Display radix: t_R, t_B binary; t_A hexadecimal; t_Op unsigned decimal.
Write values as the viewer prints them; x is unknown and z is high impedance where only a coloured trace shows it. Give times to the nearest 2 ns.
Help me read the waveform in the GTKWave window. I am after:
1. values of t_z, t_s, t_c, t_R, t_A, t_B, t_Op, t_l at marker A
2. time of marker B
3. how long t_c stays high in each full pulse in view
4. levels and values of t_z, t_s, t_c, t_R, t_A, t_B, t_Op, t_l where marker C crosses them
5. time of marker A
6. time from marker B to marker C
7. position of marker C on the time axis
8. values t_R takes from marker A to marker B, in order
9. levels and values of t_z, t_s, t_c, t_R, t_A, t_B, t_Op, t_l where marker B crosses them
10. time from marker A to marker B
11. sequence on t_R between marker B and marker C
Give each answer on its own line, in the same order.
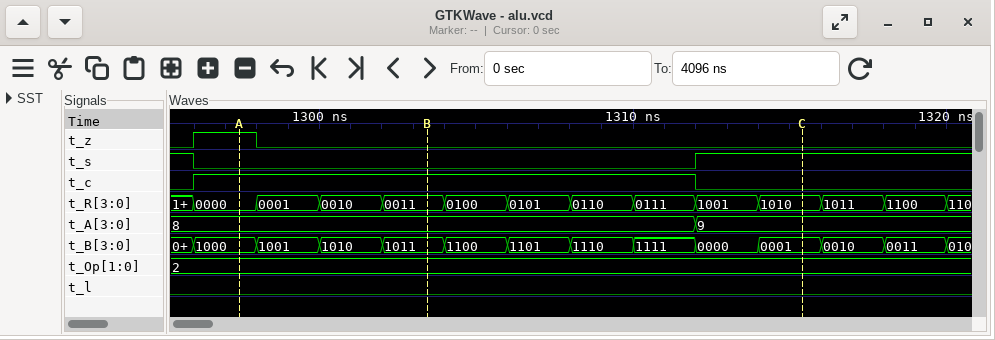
t_z=1, t_s=0, t_c=1, t_R=0000, t_A=8, t_B=1000, t_Op=2, t_l=0
1304 ns
16 ns
t_z=0, t_s=1, t_c=0, t_R=1010, t_A=9, t_B=0001, t_Op=2, t_l=0
1298 ns
12 ns
1316 ns
0000, 0001, 0010, 0011
t_z=0, t_s=0, t_c=1, t_R=0011, t_A=8, t_B=1011, t_Op=2, t_l=0
6 ns
0011, 0100, 0101, 0110, 0111, 1001, 1010
